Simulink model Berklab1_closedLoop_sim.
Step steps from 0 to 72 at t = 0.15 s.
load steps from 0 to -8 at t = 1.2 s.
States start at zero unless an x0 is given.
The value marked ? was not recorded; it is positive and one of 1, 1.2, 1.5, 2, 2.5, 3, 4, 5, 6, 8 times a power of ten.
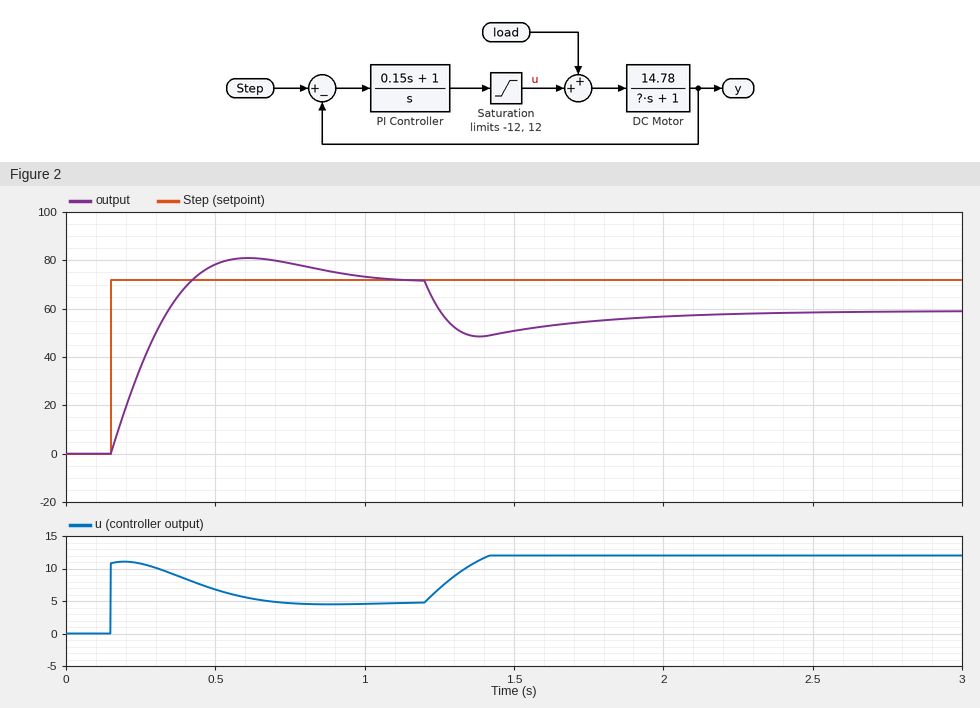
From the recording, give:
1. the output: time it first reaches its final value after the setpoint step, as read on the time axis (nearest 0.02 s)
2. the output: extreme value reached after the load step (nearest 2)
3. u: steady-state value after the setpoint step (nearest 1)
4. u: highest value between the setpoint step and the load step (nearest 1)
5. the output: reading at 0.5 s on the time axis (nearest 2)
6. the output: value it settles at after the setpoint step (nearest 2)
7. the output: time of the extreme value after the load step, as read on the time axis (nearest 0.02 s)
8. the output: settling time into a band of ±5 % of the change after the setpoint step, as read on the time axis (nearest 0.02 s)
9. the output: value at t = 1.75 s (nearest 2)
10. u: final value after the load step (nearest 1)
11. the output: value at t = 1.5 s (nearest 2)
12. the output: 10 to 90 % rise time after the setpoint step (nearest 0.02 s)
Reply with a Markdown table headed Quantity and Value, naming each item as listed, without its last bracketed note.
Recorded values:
| Quantity | Value |
|---|---|
| the output: time it first reaches its final value after the setpoint step, as read on the time axis | 0.42 s |
| the output: extreme value reached after the load step | 48 |
| u: steady-state value after the setpoint step | 5 |
| u: highest value between the setpoint step and the load step | 11 |
| the output: reading at 0.5 s on the time axis | 78 |
| the output: value it settles at after the setpoint step | 72 |
| the output: time of the extreme value after the load step, as read on the time axis | 1.38 s |
| the output: settling time into a band of ±5 % of the change after the setpoint step, as read on the time axis | 0.88 s |
| the output: value at t = 1.75 s | 54 |
| u: final value after the load step | 12 |
| the output: value at t = 1.5 s | 50 |
| the output: 10 to 90 % rise time after the setpoint step | 0.20 s |
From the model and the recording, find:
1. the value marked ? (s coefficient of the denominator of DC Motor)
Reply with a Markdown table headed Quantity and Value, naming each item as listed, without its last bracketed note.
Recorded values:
| Quantity | Value |
|---|---|
| the value marked ? | 0.4 |
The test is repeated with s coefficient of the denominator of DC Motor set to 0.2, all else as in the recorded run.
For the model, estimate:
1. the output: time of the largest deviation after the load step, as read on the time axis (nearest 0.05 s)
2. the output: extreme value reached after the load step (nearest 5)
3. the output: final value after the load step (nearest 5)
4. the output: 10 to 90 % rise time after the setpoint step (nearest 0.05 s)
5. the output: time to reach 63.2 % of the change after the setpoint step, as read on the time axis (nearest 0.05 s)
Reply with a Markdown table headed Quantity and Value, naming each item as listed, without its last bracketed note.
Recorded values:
| Quantity | Value |
|---|---|
| the output: time of the largest deviation after the load step, as read on the time axis | 1.30 s |
| the output: extreme value reached after the load step | 45 |
| the output: final value after the load step | 60 |
| the output: 10 to 90 % rise time after the setpoint step | 0.15 s |
| the output: time to reach 63.2 % of the change after the setpoint step, as read on the time axis | 0.25 s |
